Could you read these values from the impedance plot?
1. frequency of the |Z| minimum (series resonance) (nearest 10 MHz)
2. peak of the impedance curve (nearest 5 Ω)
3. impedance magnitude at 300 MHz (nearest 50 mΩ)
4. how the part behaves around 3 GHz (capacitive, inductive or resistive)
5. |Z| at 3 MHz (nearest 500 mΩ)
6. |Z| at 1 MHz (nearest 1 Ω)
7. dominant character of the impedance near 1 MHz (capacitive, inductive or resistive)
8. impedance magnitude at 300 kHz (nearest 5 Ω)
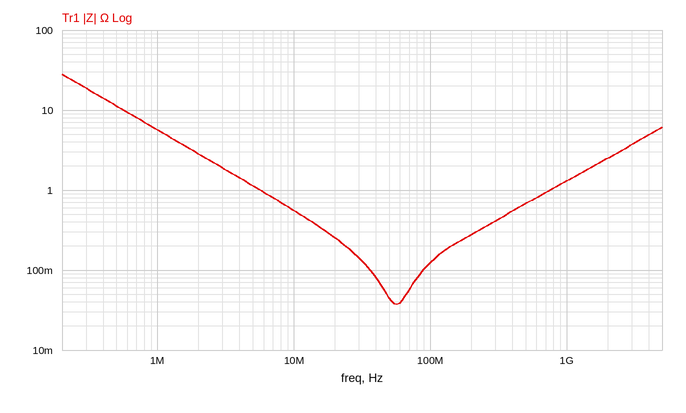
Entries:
60 MHz
30 Ω
400 mΩ
inductive
2.0 Ω
6 Ω
capacitive
20 Ω
